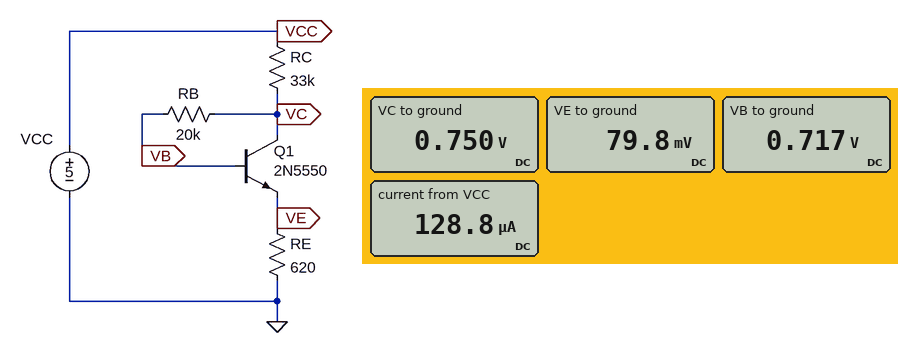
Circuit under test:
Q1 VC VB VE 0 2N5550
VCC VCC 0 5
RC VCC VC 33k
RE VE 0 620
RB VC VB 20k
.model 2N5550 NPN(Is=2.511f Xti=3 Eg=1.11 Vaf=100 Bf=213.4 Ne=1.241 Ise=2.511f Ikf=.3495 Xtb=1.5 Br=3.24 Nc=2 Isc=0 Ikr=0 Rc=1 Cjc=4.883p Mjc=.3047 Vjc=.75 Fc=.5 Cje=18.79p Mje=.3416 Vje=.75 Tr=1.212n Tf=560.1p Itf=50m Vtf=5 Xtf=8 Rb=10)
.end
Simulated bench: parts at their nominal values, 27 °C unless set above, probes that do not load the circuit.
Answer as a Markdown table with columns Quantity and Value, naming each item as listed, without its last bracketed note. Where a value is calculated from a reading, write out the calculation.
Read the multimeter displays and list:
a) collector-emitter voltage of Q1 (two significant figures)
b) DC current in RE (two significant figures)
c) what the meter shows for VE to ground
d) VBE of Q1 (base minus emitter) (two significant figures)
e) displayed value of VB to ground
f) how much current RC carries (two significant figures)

| Quantity | Value |
|---|---|
| collector-emitter voltage of Q1 | 750 mV - 79.8 mV = 670 mV |
| DC current in RE | (79.8 mV) / 620 Ω = 130 µA |
| what the meter shows for VE to ground | 79.8 mV |
| VBE of Q1 (base minus emitter) | 717 mV - 79.8 mV = 640 mV |
| displayed value of VB to ground | 0.717 V |
| how much current RC carries | (5 V - 750 mV) / 33 kΩ = 130 µA |
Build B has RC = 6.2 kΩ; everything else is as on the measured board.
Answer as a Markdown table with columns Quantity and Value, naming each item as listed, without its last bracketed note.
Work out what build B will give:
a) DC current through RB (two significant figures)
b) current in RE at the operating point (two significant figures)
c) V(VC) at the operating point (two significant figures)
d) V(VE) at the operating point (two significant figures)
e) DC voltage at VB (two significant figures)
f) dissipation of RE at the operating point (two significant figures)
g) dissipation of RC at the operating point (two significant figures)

| Quantity | Value |
|---|---|
| DC current through RB | 6.6 µA |
| current in RE at the operating point | 610 µA |
| V(VC) at the operating point | 1.2 V |
| V(VE) at the operating point | 380 mV |
| DC voltage at VB | 1.1 V |
| dissipation of RE at the operating point | 230 µW |
| dissipation of RC at the operating point | 2.3 mW |
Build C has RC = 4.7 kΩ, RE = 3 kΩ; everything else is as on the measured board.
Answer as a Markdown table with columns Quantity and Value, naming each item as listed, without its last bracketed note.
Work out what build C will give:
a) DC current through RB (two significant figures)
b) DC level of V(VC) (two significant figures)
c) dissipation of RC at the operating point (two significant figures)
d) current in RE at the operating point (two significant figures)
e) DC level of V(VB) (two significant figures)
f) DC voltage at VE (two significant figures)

| Quantity | Value |
|---|---|
| DC current through RB | 5.9 µA |
| DC level of V(VC) | 2.4 V |
| dissipation of RC at the operating point | 1.4 mW |
| current in RE at the operating point | 550 µA |
| DC level of V(VB) | 2.3 V |
| DC voltage at VE | 1.6 V |
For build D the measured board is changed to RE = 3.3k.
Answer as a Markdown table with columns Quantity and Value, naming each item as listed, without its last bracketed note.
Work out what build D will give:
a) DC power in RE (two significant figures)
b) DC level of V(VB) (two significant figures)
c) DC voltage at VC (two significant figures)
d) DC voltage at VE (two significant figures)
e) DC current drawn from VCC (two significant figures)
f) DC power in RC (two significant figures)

| Quantity | Value |
|---|---|
| DC power in RE | 47 µW |
| DC level of V(VB) | 1.0 V |
| DC voltage at VC | 1.1 V |
| DC voltage at VE | 390 mV |
| DC current drawn from VCC | 120 µA |
| DC power in RC | 470 µW |
